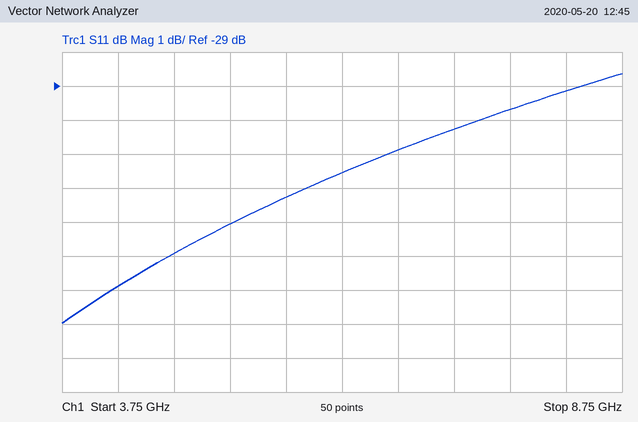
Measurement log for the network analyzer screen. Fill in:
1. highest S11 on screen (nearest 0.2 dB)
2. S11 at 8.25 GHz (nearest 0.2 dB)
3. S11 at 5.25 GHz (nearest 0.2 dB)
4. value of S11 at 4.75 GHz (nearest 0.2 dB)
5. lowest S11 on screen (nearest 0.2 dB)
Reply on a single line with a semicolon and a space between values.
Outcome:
-28.6 dB; -29.2 dB; -33.0 dB; -34.0 dB; -36.0 dB
